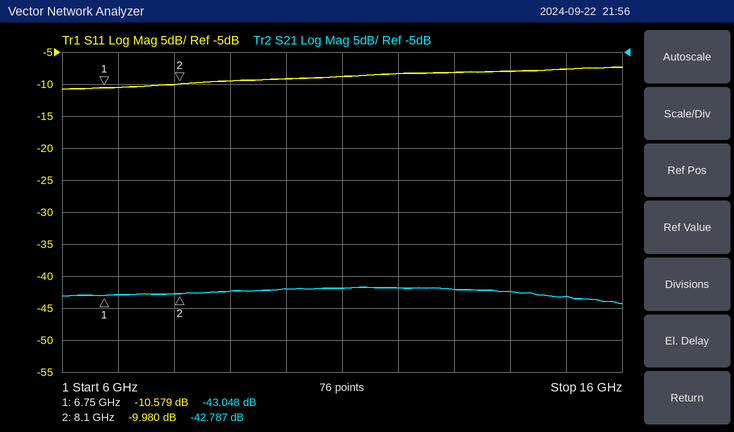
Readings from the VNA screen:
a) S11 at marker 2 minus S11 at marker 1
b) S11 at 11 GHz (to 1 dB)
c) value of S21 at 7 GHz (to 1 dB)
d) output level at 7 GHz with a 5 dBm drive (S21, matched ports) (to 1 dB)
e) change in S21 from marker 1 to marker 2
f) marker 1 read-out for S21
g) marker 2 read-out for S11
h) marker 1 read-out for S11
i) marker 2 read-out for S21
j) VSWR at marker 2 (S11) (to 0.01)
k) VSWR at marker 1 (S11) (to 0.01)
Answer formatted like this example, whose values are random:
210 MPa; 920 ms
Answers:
0.599 dB; -9 dB; -43 dB; -38 dBm; 0.261 dB; -43.048 dB; -9.980 dB; -10.579 dB; -42.787 dB; 1.93; 1.84
